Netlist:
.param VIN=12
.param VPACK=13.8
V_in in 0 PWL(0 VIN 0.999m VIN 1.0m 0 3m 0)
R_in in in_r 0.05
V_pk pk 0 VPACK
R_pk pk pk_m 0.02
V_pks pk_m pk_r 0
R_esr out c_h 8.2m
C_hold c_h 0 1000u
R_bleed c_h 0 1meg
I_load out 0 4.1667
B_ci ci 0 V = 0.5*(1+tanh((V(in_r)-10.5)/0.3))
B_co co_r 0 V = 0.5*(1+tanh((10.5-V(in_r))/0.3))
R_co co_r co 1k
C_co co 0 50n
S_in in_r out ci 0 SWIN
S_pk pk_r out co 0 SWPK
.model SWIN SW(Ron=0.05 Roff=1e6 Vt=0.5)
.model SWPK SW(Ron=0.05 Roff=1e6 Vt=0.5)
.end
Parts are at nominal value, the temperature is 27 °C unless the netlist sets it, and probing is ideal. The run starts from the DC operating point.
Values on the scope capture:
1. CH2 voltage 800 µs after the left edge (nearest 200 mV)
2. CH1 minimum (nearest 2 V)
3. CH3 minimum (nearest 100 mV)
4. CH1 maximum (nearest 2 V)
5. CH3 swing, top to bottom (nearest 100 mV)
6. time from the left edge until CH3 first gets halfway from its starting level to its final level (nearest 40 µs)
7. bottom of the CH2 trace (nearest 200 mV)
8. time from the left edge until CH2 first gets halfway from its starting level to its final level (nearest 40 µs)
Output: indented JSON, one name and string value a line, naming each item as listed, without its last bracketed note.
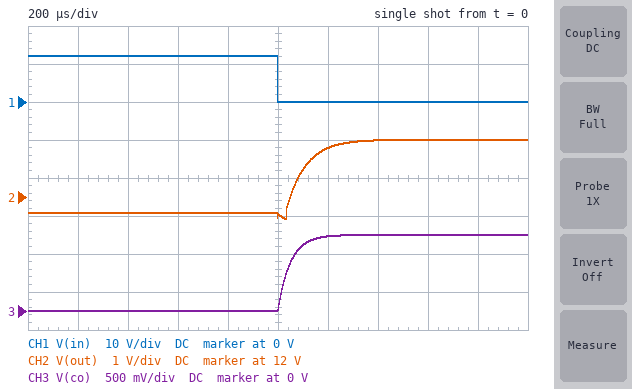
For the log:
{
  "CH2 voltage 800 µs after the left edge": "11.6 V",
  "CH1 minimum": "0 V",
  "CH3 minimum": "0 V",
  "CH1 maximum": "12 V",
  "CH3 swing, top to bottom": "1.0 V",
  "time from the left edge until CH3 first gets halfway from its starting level to its final level": "1.04 ms",
  "bottom of the CH2 trace": "11.4 V",
  "time from the left edge until CH2 first gets halfway from its starting level to its final level": "1.08 ms"
}
